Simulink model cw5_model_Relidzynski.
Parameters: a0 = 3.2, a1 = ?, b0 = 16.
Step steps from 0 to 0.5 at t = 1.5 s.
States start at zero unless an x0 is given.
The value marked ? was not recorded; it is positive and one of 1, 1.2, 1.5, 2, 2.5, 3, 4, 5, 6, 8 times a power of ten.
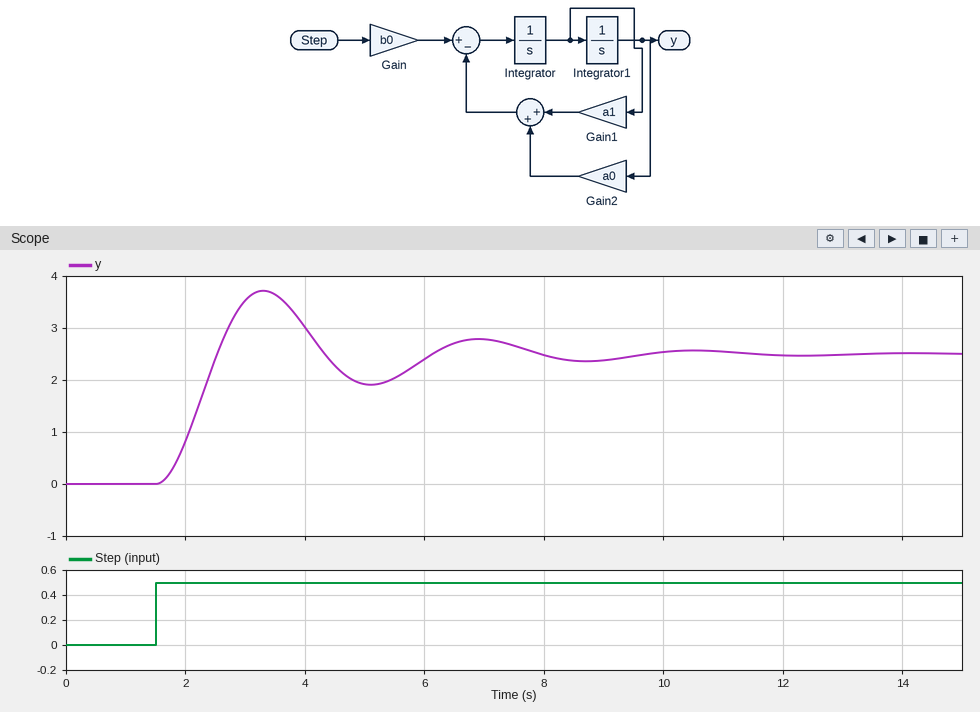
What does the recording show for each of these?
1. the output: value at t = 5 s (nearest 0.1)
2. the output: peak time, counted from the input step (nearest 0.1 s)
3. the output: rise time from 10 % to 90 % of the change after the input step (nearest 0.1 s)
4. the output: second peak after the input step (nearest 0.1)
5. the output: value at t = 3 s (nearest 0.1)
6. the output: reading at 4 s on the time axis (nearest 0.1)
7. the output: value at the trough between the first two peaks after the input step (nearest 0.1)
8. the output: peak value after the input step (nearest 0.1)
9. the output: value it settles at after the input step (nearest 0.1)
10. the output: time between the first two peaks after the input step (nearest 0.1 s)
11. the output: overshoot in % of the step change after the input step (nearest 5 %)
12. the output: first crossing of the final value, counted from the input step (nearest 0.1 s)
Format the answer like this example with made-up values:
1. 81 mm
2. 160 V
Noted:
1. 1.9
2. 1.8 s
3. 0.7 s
4. 2.8
5. 3.5
6. 3.0
7. 1.9
8. 3.7
9. 2.5
10. 3.6 s
11. 50 %
12. 1.0 s
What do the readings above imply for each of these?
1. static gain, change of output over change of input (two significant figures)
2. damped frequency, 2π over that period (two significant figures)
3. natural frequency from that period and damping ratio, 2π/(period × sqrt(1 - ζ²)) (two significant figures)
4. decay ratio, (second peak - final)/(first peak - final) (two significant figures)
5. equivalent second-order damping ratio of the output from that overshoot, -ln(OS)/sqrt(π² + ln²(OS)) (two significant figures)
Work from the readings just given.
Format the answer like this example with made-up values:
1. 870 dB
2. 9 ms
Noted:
1. 5.0
2. 1.7 rad/s
3. 1.8 rad/s
4. 0.25
5. 0.22
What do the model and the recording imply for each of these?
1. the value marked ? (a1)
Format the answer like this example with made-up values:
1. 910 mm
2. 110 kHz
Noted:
1. 0.8
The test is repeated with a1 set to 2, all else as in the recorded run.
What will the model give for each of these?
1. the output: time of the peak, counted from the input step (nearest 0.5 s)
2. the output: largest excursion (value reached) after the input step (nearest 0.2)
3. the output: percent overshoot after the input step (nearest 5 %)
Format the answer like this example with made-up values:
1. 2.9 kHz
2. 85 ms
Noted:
1. 2.0 s
2. 2.8
3. 10 %
